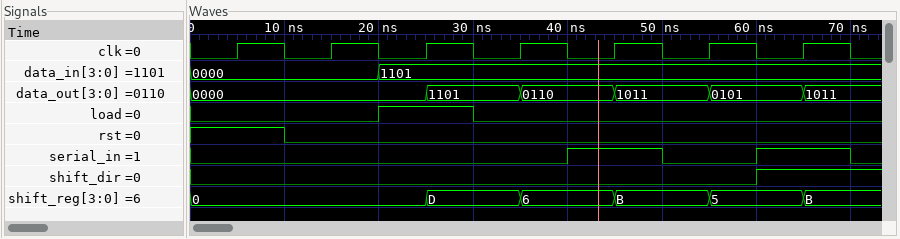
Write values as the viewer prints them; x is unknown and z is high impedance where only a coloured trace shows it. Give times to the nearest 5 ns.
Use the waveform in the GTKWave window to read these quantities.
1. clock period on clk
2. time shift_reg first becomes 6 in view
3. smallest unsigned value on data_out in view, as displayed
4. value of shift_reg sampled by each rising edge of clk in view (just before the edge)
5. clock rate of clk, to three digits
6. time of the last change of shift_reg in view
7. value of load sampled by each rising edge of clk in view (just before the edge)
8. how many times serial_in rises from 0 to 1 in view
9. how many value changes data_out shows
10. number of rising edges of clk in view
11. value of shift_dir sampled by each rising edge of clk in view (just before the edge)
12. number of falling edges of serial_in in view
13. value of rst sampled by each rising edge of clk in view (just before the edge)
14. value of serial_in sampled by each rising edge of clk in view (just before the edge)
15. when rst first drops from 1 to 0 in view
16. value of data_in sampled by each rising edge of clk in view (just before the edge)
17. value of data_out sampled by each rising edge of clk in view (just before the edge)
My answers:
10 ns
35 ns
0000
0, 0, 0, D, 6, B, 5
100 MHz
65 ns
0 0 1 0 0 0 0
2
5
7
0 0 0 0 0 0 1
2
1 0 0 0 0 0 0
0 0 0 0 1 0 1
10 ns
0000, 0000, 1101, 1101, 1101, 1101, 1101
0000, 0000, 0000, 1101, 0110, 1011, 0101
